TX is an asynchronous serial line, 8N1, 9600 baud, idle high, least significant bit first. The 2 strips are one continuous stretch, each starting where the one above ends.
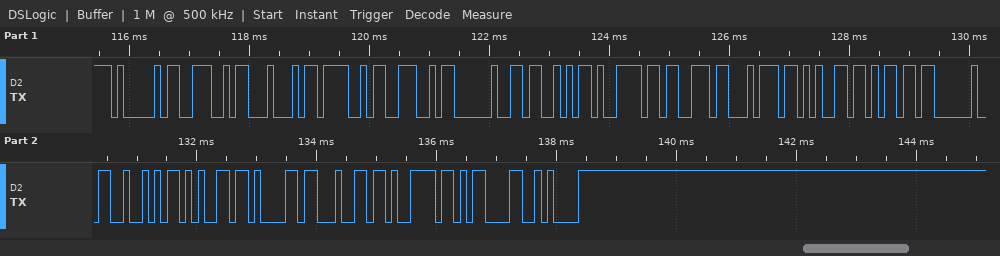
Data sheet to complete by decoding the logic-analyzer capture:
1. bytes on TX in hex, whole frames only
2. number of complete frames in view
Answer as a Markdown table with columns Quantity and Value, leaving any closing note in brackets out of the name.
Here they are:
| Quantity | Value |
|---|---|
| bytes on TX in hex, whole frames only | 41 4E 44 4F 4E 20 53 79 73 74 65 6D 20 52 65 61 64 79 0D 0A |
| number of complete frames in view | 20 |
